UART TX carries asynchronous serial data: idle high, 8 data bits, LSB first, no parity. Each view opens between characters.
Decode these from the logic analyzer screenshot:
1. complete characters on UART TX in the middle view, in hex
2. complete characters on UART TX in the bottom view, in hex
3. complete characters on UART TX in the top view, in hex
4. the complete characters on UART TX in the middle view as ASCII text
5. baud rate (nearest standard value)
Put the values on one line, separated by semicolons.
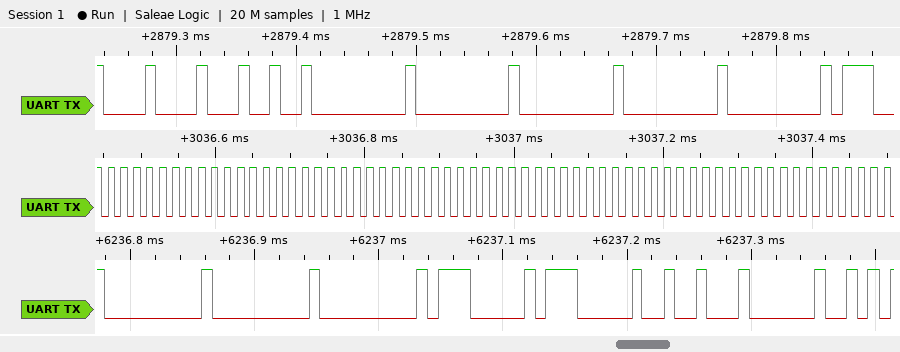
55, 55, 55, 55, 55, 55, 55, 55, 55, 55, 55, 55; 00, 00, 00, 07, 07, 12, 20; 08, 24, 00, 00, 00, 00, 00; "UUUUUUUUUUUU"; 115200 baud
